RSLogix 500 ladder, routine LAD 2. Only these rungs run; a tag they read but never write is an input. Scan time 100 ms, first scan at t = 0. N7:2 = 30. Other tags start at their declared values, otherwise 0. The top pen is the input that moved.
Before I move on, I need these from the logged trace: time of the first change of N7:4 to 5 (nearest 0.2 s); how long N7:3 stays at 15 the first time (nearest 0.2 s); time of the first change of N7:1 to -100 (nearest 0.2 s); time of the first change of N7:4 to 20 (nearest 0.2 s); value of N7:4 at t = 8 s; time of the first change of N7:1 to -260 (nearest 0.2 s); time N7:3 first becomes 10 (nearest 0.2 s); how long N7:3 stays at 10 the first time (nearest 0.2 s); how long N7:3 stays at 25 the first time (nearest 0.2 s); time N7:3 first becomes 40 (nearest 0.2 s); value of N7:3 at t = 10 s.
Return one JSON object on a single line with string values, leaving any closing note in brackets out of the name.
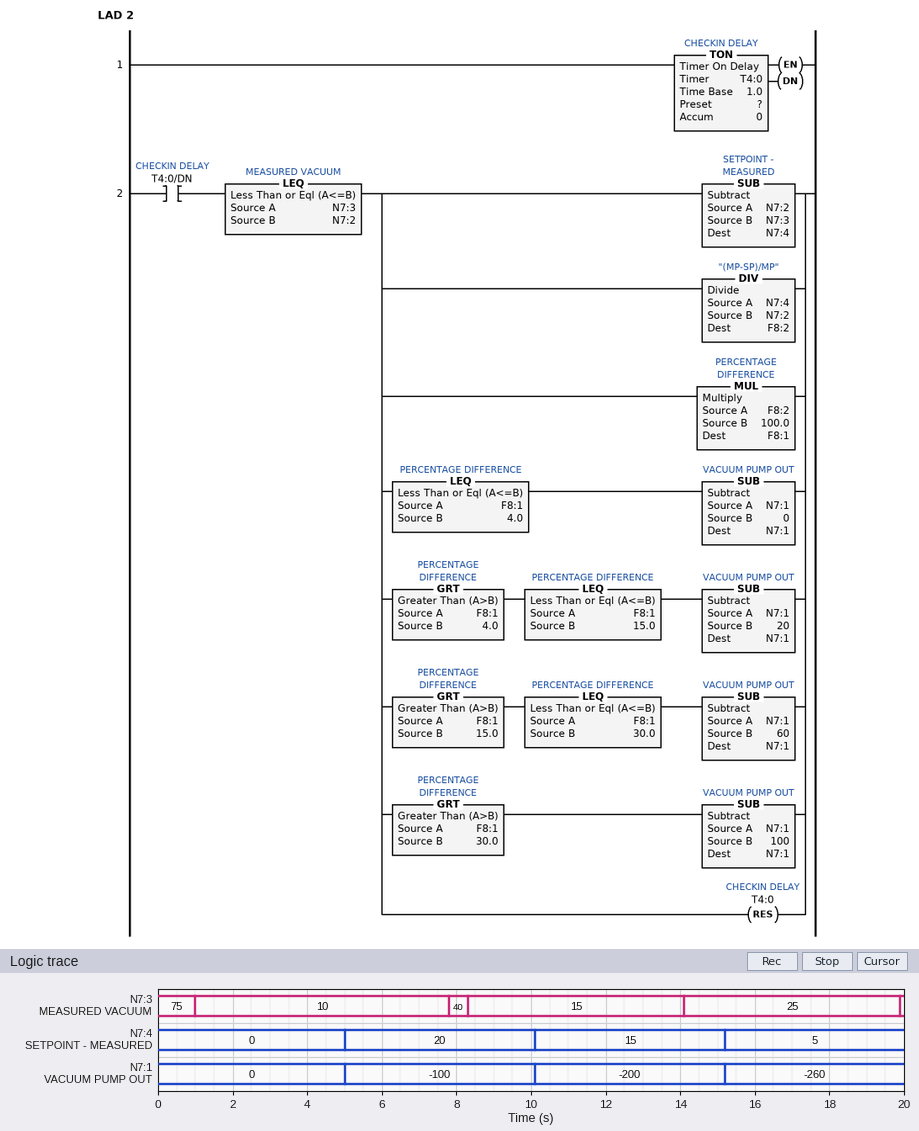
{"time of the first change of N7:4 to 5": "15.2 s", "how long N7:3 stays at 15 the first time": "5.8 s", "time of the first change of N7:1 to -100": "5.0 s", "time of the first change of N7:4 to 20": "5.0 s", "value of N7:4 at t = 8 s": "20", "time of the first change of N7:1 to -260": "15.2 s", "time N7:3 first becomes 10": "1.0 s", "how long N7:3 stays at 10 the first time": "6.8 s", "how long N7:3 stays at 25 the first time": "5.8 s", "time N7:3 first becomes 40": "7.8 s", "value of N7:3 at t = 10 s": "15"}
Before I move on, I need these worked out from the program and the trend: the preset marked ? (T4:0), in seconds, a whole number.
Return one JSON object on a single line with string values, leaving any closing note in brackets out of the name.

{"the preset marked ? (T4:0), in seconds, a whole number": "5 s"}
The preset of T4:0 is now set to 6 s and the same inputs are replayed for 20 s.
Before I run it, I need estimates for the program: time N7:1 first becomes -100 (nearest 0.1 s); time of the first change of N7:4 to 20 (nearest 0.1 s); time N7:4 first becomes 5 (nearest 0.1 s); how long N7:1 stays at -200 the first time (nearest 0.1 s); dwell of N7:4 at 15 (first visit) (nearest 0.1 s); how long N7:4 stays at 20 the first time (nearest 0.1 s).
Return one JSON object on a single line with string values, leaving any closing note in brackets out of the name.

{"time N7:1 first becomes -100": "6.0 s", "time of the first change of N7:4 to 20": "6.0 s", "time N7:4 first becomes 5": "18.2 s", "how long N7:1 stays at -200 the first time": "6.1 s", "dwell of N7:4 at 15 (first visit)": "6.1 s", "how long N7:4 stays at 20 the first time": "6.1 s"}
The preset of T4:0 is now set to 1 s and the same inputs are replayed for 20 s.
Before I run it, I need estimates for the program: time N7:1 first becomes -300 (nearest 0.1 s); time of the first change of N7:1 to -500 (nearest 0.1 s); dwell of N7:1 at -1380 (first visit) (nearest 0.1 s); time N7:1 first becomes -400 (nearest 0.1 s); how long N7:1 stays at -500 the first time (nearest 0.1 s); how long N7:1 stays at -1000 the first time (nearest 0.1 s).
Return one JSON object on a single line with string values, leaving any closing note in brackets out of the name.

{"time N7:1 first becomes -300": "3.2 s", "time of the first change of N7:1 to -500": "5.4 s", "dwell of N7:1 at -1380 (first visit)": "1.1 s", "time N7:1 first becomes -400": "4.3 s", "how long N7:1 stays at -500 the first time": "1.1 s", "how long N7:1 stays at -1000 the first time": "1.1 s"}
